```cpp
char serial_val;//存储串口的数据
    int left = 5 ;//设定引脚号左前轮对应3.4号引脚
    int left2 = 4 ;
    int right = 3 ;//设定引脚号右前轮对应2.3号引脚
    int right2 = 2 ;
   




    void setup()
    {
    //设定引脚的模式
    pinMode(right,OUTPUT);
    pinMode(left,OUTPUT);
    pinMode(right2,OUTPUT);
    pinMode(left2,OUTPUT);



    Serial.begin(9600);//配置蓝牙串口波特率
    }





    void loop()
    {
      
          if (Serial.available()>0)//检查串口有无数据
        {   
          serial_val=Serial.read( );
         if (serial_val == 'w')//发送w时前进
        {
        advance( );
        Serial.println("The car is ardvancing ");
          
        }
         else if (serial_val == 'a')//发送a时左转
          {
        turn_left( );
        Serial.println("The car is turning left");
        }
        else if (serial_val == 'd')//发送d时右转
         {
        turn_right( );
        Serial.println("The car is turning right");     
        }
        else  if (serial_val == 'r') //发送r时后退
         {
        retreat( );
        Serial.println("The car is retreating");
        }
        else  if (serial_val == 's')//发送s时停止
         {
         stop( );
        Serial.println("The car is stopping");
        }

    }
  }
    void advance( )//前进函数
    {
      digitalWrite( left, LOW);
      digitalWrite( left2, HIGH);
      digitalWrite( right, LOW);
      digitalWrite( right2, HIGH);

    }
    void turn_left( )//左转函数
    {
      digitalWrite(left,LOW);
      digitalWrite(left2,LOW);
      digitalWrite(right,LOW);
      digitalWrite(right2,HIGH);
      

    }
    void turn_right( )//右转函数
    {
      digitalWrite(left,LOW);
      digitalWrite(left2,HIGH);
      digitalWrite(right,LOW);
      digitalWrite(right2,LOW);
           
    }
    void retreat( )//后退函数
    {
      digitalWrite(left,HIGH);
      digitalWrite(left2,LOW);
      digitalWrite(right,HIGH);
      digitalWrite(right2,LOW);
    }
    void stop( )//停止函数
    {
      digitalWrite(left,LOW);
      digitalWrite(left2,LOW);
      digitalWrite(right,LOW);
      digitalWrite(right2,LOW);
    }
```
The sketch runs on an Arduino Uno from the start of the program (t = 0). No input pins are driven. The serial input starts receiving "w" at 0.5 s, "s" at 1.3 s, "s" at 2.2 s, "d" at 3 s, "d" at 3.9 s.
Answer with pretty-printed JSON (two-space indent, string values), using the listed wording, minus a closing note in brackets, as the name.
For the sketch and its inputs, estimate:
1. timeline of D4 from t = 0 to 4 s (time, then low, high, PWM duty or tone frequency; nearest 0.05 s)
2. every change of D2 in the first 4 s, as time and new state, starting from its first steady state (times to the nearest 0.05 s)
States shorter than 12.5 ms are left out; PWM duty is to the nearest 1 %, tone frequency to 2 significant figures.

{
  "timeline of D4 from t = 0 to 4 s": "0 s low; 0.5 s high; 1.3 s low; 3 s high",
  "every change of D2 in the first 4 s, as time and new state, starting from its first steady state": "0 s low; 0.5 s high; 1.3 s low"
}
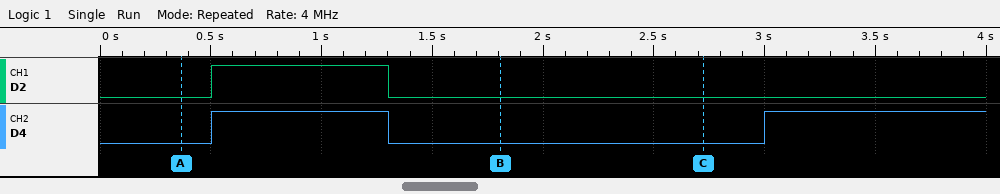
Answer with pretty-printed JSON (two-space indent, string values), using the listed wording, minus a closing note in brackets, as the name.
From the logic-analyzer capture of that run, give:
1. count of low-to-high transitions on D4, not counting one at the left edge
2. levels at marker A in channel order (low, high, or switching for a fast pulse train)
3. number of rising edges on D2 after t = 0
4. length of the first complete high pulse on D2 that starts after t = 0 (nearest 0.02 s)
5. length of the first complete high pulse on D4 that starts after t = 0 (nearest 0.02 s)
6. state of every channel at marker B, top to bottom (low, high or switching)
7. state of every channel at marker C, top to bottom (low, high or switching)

{
  "count of low-to-high transitions on D4, not counting one at the left edge": "2",
  "levels at marker A in channel order": "D2 low, D4 low",
  "number of rising edges on D2 after t = 0": "1",
  "length of the first complete high pulse on D2 that starts after t = 0": "0.80 s",
  "length of the first complete high pulse on D4 that starts after t = 0": "0.80 s",
  "state of every channel at marker B, top to bottom": "D2 low, D4 low",
  "state of every channel at marker C, top to bottom": "D2 low, D4 low"
}
